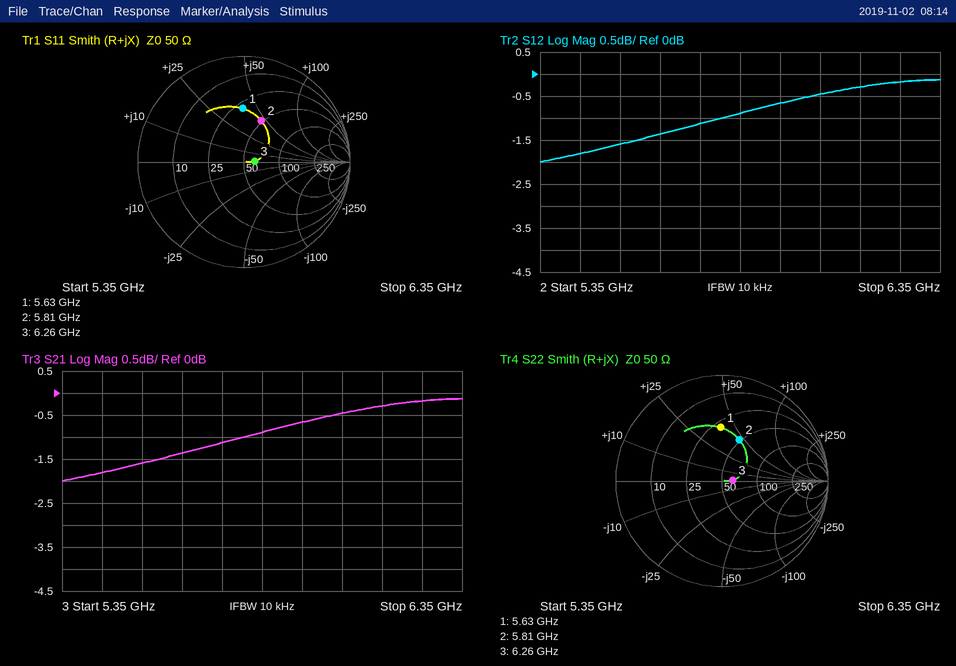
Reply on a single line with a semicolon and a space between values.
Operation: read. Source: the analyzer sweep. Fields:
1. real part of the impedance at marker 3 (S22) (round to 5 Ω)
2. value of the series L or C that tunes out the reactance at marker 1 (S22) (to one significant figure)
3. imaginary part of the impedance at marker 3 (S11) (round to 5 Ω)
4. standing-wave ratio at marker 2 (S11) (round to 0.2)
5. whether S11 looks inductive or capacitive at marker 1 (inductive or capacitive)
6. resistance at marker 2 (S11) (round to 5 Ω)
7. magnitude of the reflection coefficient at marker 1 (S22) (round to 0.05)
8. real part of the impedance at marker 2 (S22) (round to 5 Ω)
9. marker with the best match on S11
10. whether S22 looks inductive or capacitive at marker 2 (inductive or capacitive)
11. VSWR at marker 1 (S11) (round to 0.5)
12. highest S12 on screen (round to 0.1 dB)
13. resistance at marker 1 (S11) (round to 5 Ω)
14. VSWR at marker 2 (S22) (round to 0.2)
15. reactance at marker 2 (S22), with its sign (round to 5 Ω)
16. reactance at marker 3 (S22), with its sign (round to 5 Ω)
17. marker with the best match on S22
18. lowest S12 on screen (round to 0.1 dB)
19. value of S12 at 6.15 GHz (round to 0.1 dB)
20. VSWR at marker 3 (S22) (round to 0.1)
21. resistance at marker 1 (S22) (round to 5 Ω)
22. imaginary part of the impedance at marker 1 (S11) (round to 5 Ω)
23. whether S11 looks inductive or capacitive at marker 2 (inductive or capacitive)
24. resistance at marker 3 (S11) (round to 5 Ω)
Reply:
60 Ω; 700 fF; 0 Ω; 2.4; inductive; 50 Ω; 0.50; 50 Ω; marker 3; inductive; 3.0; -0.1 dB; 30 Ω; 2.4; +45 Ω; 0 Ω; marker 3; -2.0 dB; -0.3 dB; 1.2; 30 Ω; +40 Ω; inductive; 60 Ω
